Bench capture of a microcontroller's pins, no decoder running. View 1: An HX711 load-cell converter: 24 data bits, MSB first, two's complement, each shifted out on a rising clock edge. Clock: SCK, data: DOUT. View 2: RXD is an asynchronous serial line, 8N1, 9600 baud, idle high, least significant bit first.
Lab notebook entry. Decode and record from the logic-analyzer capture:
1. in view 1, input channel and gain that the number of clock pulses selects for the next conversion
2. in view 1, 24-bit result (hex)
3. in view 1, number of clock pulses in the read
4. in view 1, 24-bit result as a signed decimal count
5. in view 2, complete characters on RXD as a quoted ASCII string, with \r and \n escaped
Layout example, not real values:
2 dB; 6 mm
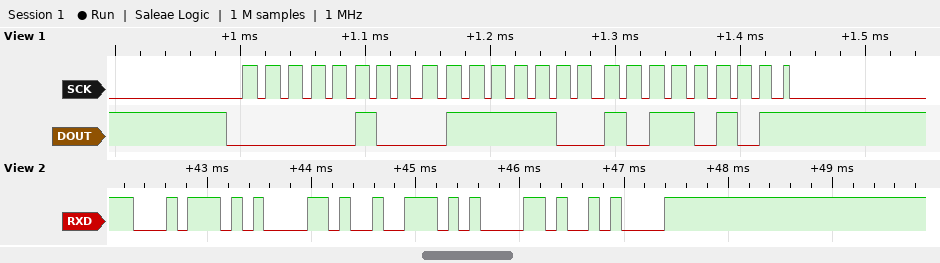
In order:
channel A, gain 128; 0x047CB5; 25; 294069; "tara\n"
